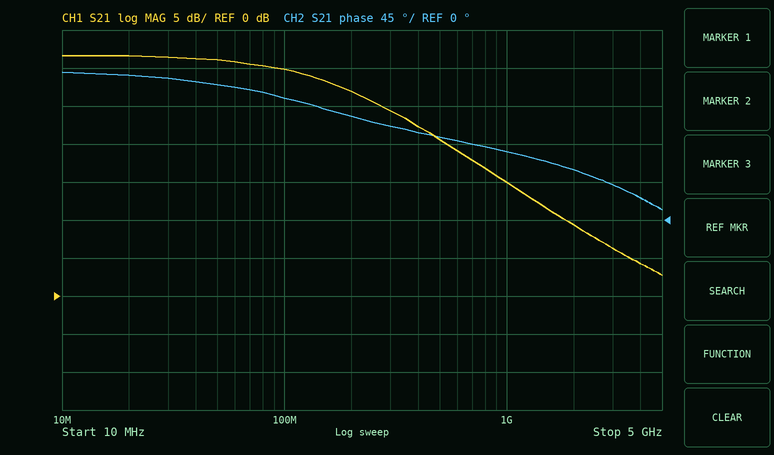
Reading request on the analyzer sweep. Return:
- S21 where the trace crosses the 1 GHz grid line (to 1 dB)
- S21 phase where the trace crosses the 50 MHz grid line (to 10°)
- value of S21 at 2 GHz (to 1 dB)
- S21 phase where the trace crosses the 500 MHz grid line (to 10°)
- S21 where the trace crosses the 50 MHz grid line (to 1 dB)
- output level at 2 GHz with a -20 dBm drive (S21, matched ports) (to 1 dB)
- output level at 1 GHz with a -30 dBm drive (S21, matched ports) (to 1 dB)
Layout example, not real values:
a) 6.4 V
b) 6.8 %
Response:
a) 15 dB
b) 160°
c) 9 dB
d) 100°
e) 31 dB
f) -11 dBm
g) -15 dBm
